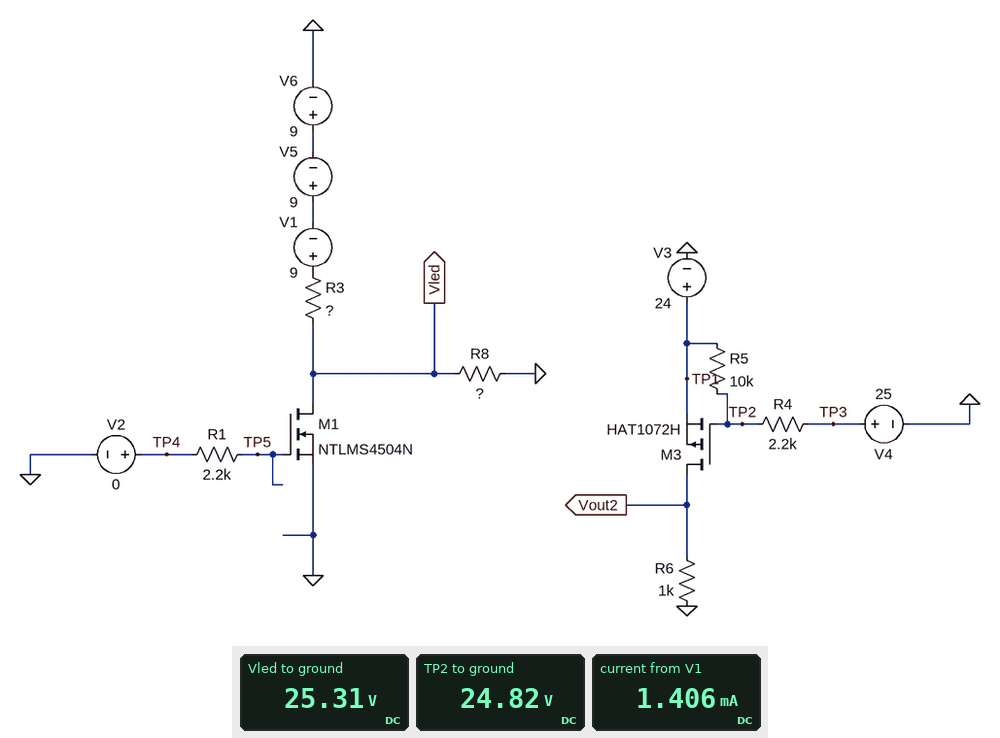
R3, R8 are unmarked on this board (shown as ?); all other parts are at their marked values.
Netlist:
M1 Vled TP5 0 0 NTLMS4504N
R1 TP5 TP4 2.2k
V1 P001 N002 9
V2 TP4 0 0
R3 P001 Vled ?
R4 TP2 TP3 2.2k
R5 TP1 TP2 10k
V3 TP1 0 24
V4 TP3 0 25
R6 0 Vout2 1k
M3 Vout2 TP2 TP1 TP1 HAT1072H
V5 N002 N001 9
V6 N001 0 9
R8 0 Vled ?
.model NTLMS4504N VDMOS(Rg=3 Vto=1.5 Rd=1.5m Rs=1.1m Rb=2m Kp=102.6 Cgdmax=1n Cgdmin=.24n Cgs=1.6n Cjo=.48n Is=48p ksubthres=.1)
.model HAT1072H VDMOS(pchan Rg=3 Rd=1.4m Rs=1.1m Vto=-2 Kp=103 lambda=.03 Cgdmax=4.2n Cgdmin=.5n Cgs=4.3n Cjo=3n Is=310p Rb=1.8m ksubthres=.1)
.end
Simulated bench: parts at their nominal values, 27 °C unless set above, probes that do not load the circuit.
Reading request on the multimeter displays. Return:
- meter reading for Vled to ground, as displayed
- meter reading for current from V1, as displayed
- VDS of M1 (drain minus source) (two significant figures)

25.31 V
1.406 mA
25 V
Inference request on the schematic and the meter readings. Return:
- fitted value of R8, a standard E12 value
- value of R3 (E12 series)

18 kΩ
1.2 kΩ
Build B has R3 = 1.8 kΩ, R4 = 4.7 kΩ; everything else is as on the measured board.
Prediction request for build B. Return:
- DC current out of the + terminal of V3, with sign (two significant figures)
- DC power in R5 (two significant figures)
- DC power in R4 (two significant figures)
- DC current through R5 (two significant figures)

-68 µA
46 µW
22 µW
68 µA
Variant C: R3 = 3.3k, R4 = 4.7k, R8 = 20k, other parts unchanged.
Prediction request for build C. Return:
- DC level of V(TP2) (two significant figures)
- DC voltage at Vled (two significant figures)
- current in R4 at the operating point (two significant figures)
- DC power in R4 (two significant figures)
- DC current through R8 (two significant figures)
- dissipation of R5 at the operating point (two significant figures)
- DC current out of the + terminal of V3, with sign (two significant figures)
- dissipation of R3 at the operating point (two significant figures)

25 V
23 V
68 µA
22 µW
1.2 mA
46 µW
-68 µA
4.4 mW
